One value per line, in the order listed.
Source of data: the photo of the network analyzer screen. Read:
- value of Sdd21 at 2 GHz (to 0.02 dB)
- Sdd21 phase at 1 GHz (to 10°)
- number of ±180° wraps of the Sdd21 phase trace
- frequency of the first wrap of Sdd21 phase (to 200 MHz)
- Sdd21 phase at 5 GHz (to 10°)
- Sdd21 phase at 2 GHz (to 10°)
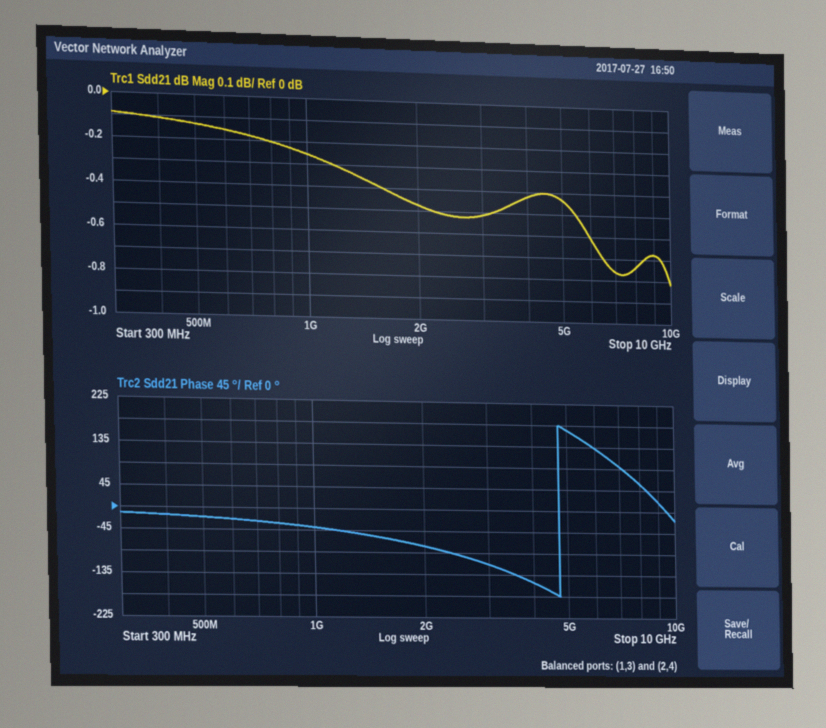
-0.48 dB
-40°
1
4.8 GHz
170°
-80°
